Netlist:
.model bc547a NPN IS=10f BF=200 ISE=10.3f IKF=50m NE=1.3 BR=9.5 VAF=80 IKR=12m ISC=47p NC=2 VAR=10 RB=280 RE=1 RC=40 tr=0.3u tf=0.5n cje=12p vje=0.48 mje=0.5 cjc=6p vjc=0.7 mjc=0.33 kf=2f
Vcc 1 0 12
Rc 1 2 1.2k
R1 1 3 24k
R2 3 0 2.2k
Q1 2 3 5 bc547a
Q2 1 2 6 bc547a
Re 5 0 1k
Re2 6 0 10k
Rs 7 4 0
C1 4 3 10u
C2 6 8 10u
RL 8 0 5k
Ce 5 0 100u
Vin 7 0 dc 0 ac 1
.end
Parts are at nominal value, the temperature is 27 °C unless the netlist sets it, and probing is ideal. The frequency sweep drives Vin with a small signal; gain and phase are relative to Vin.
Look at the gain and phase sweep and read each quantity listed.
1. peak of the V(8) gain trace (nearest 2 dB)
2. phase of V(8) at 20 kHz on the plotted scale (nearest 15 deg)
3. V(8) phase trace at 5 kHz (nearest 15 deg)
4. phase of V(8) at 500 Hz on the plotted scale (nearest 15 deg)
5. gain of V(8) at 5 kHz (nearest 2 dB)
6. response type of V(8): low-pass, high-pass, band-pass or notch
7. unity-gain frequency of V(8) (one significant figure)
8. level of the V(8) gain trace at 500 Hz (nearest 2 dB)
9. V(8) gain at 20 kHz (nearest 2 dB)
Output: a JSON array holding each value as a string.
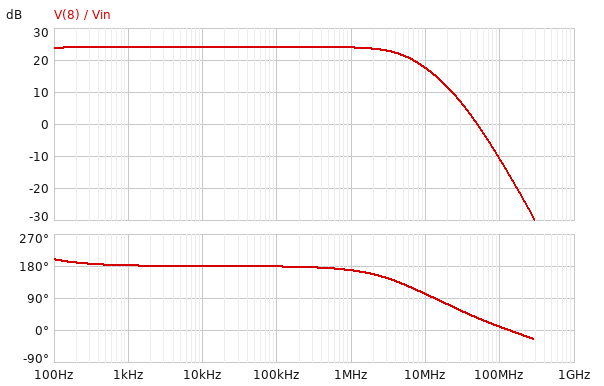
["24 dB", "180 deg", "180 deg", "180 deg", "24 dB", "low-pass", "50 MHz", "24 dB", "24 dB"]
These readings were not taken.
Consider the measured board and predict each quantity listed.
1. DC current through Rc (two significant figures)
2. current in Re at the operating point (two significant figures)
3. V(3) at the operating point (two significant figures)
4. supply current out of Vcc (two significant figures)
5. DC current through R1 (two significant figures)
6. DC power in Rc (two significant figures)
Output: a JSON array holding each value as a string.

["380 µA", "370 µA", "1.0 V", "1.9 mA", "460 µA", "170 µW"]
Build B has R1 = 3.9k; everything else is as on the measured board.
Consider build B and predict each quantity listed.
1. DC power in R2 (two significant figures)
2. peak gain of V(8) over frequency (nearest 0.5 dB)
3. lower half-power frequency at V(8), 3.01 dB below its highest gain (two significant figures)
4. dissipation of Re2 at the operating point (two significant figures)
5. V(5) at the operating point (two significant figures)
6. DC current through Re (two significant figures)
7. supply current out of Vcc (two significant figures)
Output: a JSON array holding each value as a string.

["8.4 mW", "40.0 dB", "150 Hz", "5.0 mW", "3.6 V", "3.6 mA", "6.2 mA"]
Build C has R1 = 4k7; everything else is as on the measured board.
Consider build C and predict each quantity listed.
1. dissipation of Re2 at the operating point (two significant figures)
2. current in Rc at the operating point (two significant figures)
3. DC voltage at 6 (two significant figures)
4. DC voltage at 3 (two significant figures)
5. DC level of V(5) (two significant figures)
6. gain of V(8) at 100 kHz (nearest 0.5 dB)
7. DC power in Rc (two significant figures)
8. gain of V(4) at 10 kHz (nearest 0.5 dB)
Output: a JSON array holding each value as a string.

["5.9 mW", "3.1 mA", "7.7 V", "3.8 V", "3.1 V", "39.5 dB", "11 mW", "0 dB"]
